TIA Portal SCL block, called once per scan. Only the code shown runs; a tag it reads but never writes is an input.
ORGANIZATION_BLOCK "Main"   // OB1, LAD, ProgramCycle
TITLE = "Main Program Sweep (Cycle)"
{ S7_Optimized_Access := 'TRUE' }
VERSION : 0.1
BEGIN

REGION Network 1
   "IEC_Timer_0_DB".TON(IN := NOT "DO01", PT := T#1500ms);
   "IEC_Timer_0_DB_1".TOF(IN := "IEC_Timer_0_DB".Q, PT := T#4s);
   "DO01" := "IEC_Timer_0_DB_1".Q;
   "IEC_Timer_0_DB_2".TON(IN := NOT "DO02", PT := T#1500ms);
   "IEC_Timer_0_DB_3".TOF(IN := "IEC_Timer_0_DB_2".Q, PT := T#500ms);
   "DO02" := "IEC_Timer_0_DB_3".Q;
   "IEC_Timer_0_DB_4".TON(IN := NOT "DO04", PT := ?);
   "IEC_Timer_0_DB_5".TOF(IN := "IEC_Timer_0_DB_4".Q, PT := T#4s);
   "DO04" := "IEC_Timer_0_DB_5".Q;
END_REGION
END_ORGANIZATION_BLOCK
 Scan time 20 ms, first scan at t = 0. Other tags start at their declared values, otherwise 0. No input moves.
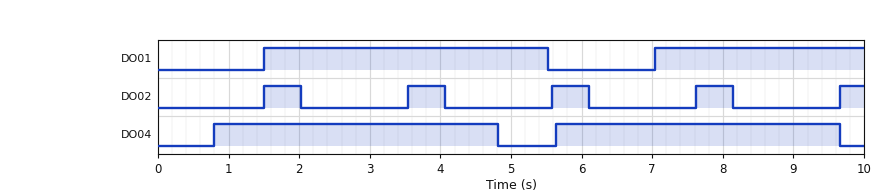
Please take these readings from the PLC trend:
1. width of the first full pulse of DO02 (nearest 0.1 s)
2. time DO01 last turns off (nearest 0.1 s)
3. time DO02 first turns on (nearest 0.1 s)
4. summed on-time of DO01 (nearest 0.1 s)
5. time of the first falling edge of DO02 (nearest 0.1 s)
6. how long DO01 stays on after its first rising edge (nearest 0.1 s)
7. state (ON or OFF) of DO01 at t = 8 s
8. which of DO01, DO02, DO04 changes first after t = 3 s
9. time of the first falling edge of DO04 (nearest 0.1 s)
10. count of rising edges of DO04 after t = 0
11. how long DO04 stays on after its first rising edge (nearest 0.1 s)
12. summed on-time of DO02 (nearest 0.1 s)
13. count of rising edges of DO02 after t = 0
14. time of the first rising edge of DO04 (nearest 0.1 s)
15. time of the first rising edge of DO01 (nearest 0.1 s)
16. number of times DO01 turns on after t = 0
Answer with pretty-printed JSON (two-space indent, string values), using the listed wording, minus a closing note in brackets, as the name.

{
  "width of the first full pulse of DO02": "0.5 s",
  "time DO01 last turns off": "5.5 s",
  "time DO02 first turns on": "1.5 s",
  "summed on-time of DO01": "7.0 s",
  "time of the first falling edge of DO02": "2.0 s",
  "how long DO01 stays on after its first rising edge": "4.0 s",
  "state (ON or OFF) of DO01 at t = 8 s": "ON",
  "which of DO01, DO02, DO04 changes first after t = 3 s": "DO02",
  "time of the first falling edge of DO04": "4.8 s",
  "count of rising edges of DO04 after t = 0": "2",
  "how long DO04 stays on after its first rising edge": "4.0 s",
  "summed on-time of DO02": "2.4 s",
  "count of rising edges of DO02 after t = 0": "5",
  "time of the first rising edge of DO04": "0.8 s",
  "time of the first rising edge of DO01": "1.5 s",
  "number of times DO01 turns on after t = 0": "2"
}
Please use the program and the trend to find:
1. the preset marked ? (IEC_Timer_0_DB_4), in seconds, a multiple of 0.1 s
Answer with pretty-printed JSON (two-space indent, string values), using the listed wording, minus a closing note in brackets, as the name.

{
  "the preset marked ? (IEC_Timer_0_DB_4), in seconds, a multiple of 0.1 s": "0.8 s"
}
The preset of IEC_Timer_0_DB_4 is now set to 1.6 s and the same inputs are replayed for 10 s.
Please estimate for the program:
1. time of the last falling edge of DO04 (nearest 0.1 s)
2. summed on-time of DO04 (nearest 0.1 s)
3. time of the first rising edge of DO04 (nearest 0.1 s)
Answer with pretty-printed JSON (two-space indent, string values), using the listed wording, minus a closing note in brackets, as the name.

{
  "time of the last falling edge of DO04": "5.6 s",
  "summed on-time of DO04": "6.8 s",
  "time of the first rising edge of DO04": "1.6 s"
}
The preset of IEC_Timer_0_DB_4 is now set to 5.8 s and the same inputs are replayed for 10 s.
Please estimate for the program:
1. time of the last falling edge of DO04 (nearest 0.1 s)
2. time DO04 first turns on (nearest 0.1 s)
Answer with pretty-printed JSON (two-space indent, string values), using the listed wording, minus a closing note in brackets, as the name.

{
  "time of the last falling edge of DO04": "9.8 s",
  "time DO04 first turns on": "5.8 s"
}
